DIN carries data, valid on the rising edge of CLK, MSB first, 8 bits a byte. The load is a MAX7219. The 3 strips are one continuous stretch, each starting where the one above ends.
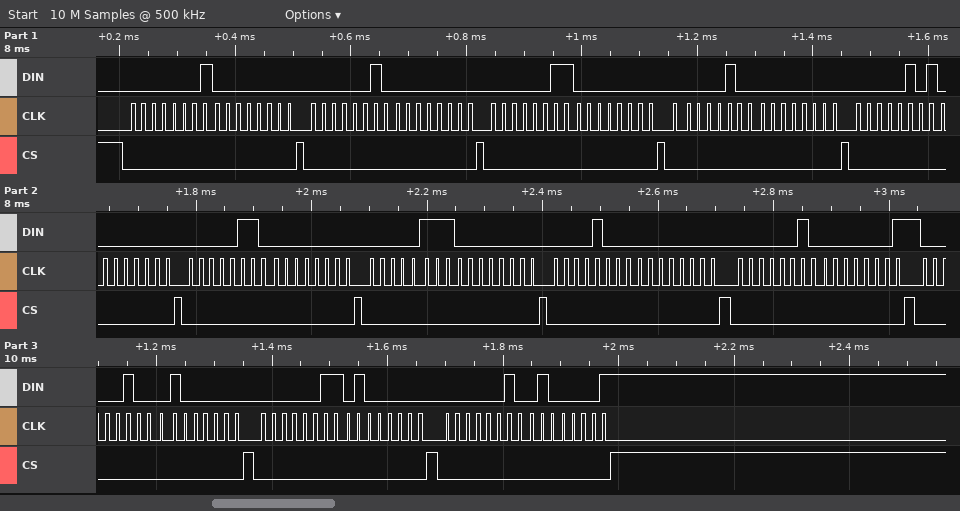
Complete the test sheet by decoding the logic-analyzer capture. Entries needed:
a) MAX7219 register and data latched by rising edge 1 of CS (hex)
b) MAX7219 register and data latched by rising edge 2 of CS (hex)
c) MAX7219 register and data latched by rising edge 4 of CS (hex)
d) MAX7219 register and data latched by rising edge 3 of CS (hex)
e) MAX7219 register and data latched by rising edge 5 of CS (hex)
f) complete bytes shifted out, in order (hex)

register 0x1, data 0x00
register 0x2, data 0x00
register 0x4, data 0x00
register 0x3, data 0x00
register 0x5, data 0x00
01 00 02 00 03 00 04 00 05 00 06 00 07 00 08 00 02 01 04 40 03 40 02 41
